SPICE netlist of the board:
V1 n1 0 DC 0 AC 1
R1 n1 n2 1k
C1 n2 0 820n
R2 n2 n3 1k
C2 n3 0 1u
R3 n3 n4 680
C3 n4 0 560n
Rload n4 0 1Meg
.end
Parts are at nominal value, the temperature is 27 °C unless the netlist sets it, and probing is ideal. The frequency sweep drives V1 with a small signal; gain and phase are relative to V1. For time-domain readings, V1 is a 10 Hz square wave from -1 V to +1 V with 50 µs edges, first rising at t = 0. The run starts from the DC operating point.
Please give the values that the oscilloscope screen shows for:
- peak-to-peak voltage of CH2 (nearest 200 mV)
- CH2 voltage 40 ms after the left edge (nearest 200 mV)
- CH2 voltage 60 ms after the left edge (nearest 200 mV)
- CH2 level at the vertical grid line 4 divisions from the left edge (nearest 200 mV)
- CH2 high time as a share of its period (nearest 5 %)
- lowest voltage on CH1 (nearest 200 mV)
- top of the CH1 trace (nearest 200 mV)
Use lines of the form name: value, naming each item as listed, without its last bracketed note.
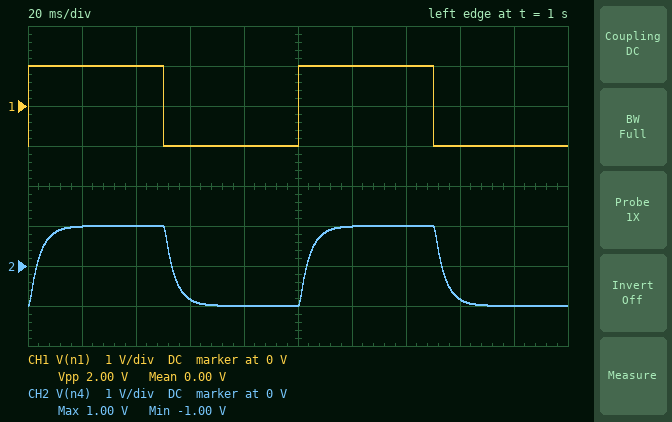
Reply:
peak-to-peak voltage of CH2: 2.0 V
CH2 voltage 40 ms after the left edge: 1.0 V
CH2 voltage 60 ms after the left edge: -800 mV
CH2 level at the vertical grid line 4 divisions from the left edge: -1.0 V
CH2 high time as a share of its period: 50 %
lowest voltage on CH1: -1.0 V
top of the CH1 trace: 1.0 V
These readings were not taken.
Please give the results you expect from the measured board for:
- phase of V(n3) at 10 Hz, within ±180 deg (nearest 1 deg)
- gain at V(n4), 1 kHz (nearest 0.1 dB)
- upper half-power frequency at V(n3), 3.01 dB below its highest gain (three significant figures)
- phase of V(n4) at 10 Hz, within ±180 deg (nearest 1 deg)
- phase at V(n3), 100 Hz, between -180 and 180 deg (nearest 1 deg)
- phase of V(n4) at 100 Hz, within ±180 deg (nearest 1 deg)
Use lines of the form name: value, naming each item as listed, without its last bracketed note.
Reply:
phase of V(n3) at 10 Hz, within ±180 deg: -14 deg
gain at V(n4), 1 kHz: -40.4 dB
upper half-power frequency at V(n3), 3.01 dB below its highest gain: 42.8 Hz
phase of V(n4) at 10 Hz, within ±180 deg: -15 deg
phase at V(n3), 100 Hz, between -180 and 180 deg: -75 deg
phase of V(n4) at 100 Hz, within ±180 deg: -88 deg
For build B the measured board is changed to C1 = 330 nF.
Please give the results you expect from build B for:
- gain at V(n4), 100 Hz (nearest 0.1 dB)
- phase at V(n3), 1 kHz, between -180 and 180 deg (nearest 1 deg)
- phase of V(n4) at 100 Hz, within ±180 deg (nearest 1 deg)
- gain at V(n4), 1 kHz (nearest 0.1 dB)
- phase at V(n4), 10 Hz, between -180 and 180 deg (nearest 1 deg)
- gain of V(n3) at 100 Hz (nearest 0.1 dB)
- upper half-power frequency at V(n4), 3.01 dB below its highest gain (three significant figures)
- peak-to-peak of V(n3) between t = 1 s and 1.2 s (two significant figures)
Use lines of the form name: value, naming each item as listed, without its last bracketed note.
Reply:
gain at V(n4), 100 Hz: -7.7 dB
phase at V(n3), 1 kHz, between -180 and 180 deg: -120 deg
phase of V(n4) at 100 Hz, within ±180 deg: -79 deg
gain at V(n4), 1 kHz: -34.8 dB
phase at V(n4), 10 Hz, between -180 and 180 deg: -14 deg
gain of V(n3) at 100 Hz: -7.4 dB
upper half-power frequency at V(n4), 3.01 dB below its highest gain: 46.1 Hz
peak-to-peak of V(n3) between t = 1 s and 1.2 s: 2.0 V
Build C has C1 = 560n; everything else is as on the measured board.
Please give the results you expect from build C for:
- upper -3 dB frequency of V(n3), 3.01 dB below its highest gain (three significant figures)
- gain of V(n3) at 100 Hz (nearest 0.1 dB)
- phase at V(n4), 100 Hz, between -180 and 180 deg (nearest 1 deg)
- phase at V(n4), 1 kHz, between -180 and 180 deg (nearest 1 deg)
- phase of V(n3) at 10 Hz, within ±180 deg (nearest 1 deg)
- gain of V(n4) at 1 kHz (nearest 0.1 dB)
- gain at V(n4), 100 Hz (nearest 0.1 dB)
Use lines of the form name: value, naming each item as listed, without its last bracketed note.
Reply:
upper -3 dB frequency of V(n3), 3.01 dB below its highest gain: 44.9 Hz
gain of V(n3) at 100 Hz: -7.8 dB
phase at V(n4), 100 Hz, between -180 and 180 deg: -84 deg
phase at V(n4), 1 kHz, between -180 and 180 deg: 159 deg
phase of V(n3) at 10 Hz, within ±180 deg: -13 deg
gain of V(n4) at 1 kHz: -37.7 dB
gain at V(n4), 100 Hz: -8.0 dB
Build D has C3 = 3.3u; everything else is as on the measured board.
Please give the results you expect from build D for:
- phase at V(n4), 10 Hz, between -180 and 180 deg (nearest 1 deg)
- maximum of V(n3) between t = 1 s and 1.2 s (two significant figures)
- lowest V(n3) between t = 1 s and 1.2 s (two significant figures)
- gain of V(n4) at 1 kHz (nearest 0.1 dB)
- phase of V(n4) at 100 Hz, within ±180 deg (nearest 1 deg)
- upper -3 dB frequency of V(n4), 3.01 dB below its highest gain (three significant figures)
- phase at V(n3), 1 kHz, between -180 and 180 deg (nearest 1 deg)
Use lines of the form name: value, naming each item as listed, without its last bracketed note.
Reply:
phase at V(n4), 10 Hz, between -180 and 180 deg: -37 deg
maximum of V(n3) between t = 1 s and 1.2 s: 980 mV
lowest V(n3) between t = 1 s and 1.2 s: -980 mV
gain of V(n4) at 1 kHz: -54.7 dB
phase of V(n4) at 100 Hz, within ±180 deg: -113 deg
upper -3 dB frequency of V(n4), 3.01 dB below its highest gain: 14.8 Hz
phase at V(n3), 1 kHz, between -180 and 180 deg: -139 deg
